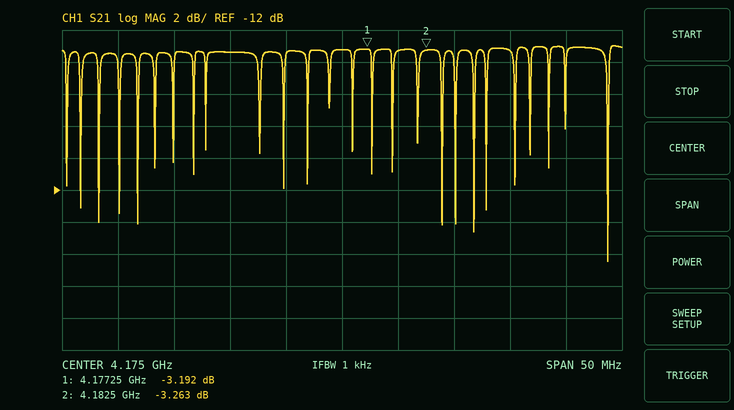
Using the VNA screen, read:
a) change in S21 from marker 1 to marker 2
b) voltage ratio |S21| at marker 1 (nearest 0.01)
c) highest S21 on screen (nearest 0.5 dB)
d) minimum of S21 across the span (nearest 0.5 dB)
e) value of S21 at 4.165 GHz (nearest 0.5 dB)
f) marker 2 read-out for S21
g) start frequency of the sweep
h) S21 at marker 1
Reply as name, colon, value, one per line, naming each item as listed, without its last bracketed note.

change in S21 from marker 1 to marker 2: -0.071 dB
voltage ratio |S21| at marker 1: 0.69
highest S21 on screen: -3.0 dB
minimum of S21 across the span: -16.5 dB
value of S21 at 4.165 GHz: -3.5 dB
marker 2 read-out for S21: -3.263 dB
start frequency of the sweep: 4.15 GHz
S21 at marker 1: -3.192 dB
